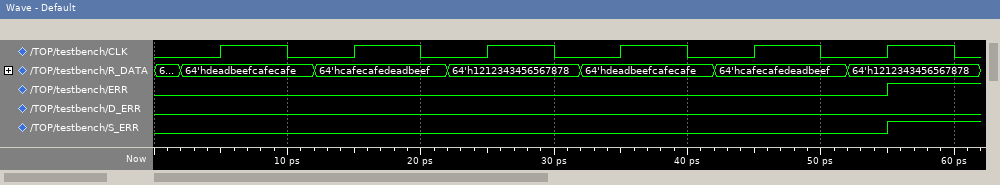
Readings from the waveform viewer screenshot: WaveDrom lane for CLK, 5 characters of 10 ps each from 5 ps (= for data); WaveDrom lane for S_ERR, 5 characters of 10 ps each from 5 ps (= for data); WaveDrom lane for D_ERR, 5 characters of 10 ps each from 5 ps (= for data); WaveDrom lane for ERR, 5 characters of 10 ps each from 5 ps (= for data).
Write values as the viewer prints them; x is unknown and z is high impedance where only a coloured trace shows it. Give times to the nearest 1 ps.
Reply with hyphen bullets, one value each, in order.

- {name: 'CLK', wave: 'p....'}
- {name: 'S_ERR', wave: '0....'}
- {name: 'D_ERR', wave: '0....'}
- {name: 'ERR', wave: '0....'}
